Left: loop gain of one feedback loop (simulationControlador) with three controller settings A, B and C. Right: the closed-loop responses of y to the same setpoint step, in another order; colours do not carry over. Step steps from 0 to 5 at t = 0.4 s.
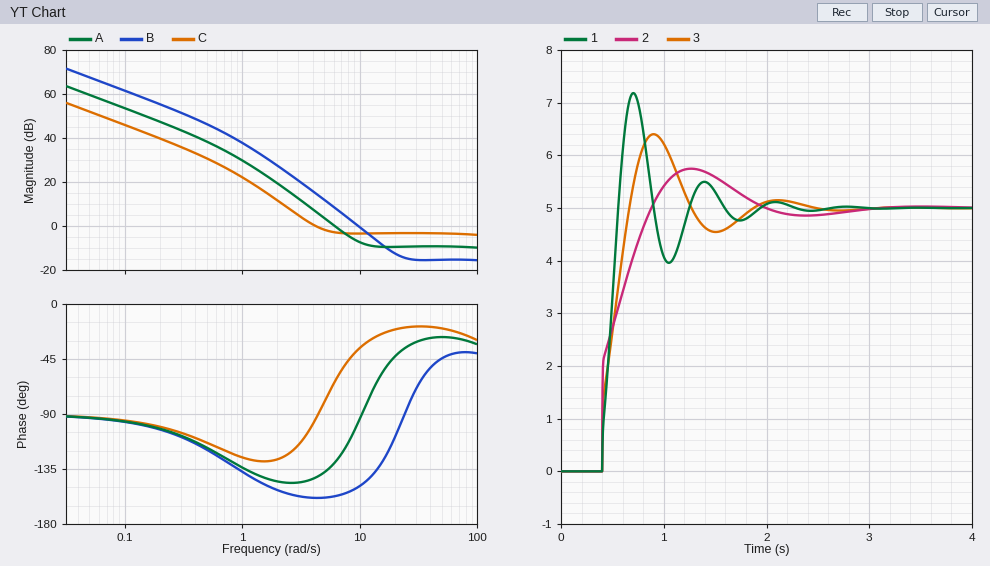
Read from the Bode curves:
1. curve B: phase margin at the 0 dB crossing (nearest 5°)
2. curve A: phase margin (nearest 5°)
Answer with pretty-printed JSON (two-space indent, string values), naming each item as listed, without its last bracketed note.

{
  "curve B: phase margin at the 0 dB crossing": "30°",
  "curve A: phase margin": "50°"
}
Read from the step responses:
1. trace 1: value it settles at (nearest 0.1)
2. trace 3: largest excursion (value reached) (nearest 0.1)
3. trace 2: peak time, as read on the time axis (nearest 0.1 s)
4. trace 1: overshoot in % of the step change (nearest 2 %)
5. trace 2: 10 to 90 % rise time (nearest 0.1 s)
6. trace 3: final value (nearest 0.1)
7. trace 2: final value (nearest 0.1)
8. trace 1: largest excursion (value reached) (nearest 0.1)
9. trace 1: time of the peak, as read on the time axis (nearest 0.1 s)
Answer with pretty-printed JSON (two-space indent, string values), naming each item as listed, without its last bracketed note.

{
  "trace 1: value it settles at": "5.0",
  "trace 3: largest excursion (value reached)": "6.4",
  "trace 2: peak time, as read on the time axis": "1.3 s",
  "trace 1: overshoot in % of the step change": "44 %",
  "trace 2: 10 to 90 % rise time": "0.4 s",
  "trace 3: final value": "5.0",
  "trace 2: final value": "5.0",
  "trace 1: largest excursion (value reached)": "7.2",
  "trace 1: time of the peak, as read on the time axis": "0.7 s"
}
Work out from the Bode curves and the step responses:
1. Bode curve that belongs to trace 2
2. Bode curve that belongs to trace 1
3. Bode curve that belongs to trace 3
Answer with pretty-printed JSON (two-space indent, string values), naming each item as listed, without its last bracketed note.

{
  "Bode curve that belongs to trace 2": "C",
  "Bode curve that belongs to trace 1": "B",
  "Bode curve that belongs to trace 3": "A"
}
